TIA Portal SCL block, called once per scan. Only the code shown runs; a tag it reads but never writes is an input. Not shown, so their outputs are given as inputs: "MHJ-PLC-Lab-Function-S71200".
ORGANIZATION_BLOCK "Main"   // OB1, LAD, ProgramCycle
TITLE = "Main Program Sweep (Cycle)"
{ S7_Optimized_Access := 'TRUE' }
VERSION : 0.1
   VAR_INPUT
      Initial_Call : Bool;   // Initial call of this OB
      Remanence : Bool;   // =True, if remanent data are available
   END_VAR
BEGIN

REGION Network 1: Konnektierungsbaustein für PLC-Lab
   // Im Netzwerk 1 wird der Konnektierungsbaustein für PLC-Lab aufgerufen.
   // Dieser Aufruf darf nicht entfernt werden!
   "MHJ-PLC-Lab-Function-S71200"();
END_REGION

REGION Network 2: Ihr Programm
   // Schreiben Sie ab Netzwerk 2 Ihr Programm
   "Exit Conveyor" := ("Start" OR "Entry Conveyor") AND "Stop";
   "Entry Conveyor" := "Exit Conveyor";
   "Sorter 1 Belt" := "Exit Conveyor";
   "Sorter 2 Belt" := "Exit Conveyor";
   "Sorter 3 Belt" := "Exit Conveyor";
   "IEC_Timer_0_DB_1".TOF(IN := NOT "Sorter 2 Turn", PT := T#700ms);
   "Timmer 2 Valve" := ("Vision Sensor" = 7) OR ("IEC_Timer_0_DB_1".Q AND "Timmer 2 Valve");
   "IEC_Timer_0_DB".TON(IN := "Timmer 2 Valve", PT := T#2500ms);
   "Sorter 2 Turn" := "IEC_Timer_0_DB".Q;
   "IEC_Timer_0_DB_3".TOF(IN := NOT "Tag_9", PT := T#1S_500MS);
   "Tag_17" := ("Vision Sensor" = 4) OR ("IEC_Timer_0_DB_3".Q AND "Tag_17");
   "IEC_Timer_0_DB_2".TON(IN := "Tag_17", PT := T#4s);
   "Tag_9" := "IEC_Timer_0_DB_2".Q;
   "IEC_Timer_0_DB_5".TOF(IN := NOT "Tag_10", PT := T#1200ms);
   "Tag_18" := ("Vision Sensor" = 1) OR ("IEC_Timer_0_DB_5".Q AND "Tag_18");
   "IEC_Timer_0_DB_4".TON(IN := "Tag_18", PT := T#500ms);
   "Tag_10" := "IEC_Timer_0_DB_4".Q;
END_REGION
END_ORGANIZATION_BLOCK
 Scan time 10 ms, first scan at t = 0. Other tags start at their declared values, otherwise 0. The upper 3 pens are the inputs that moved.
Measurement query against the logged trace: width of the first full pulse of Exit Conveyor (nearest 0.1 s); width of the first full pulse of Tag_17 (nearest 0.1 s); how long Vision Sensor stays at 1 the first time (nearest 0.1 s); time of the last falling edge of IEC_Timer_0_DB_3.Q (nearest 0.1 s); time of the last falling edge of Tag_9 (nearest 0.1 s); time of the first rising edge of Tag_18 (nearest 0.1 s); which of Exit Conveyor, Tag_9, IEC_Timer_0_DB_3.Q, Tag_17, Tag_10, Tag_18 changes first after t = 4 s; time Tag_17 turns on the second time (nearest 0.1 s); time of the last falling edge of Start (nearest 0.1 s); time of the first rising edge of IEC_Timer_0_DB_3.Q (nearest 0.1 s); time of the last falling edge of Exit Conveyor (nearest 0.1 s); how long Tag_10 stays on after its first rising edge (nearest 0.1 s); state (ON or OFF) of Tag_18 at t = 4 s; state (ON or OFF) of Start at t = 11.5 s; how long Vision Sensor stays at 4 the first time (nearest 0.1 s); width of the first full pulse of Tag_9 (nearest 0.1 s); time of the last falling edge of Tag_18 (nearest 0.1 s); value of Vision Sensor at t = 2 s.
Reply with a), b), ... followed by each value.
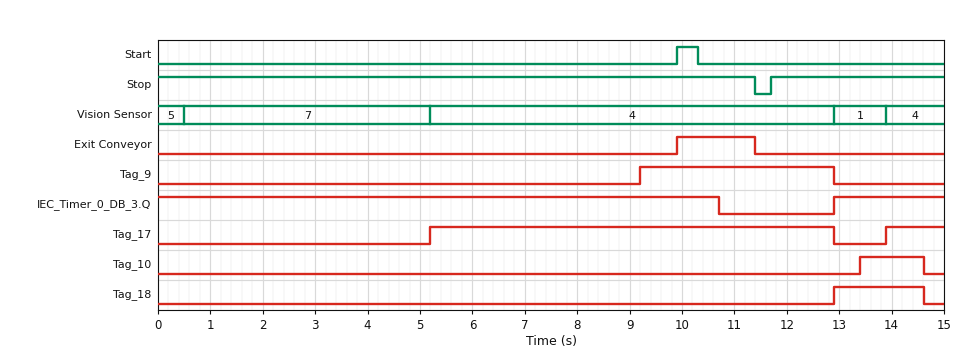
a) 1.5 s
b) 7.7 s
c) 1.0 s
d) 10.7 s
e) 12.9 s
f) 12.9 s
g) Tag_17
h) 13.9 s
i) 10.3 s
j) 12.9 s
k) 11.4 s
l) 1.2 s
m) OFF
n) OFF
o) 7.7 s
p) 3.7 s
q) 14.6 s
r) 7
